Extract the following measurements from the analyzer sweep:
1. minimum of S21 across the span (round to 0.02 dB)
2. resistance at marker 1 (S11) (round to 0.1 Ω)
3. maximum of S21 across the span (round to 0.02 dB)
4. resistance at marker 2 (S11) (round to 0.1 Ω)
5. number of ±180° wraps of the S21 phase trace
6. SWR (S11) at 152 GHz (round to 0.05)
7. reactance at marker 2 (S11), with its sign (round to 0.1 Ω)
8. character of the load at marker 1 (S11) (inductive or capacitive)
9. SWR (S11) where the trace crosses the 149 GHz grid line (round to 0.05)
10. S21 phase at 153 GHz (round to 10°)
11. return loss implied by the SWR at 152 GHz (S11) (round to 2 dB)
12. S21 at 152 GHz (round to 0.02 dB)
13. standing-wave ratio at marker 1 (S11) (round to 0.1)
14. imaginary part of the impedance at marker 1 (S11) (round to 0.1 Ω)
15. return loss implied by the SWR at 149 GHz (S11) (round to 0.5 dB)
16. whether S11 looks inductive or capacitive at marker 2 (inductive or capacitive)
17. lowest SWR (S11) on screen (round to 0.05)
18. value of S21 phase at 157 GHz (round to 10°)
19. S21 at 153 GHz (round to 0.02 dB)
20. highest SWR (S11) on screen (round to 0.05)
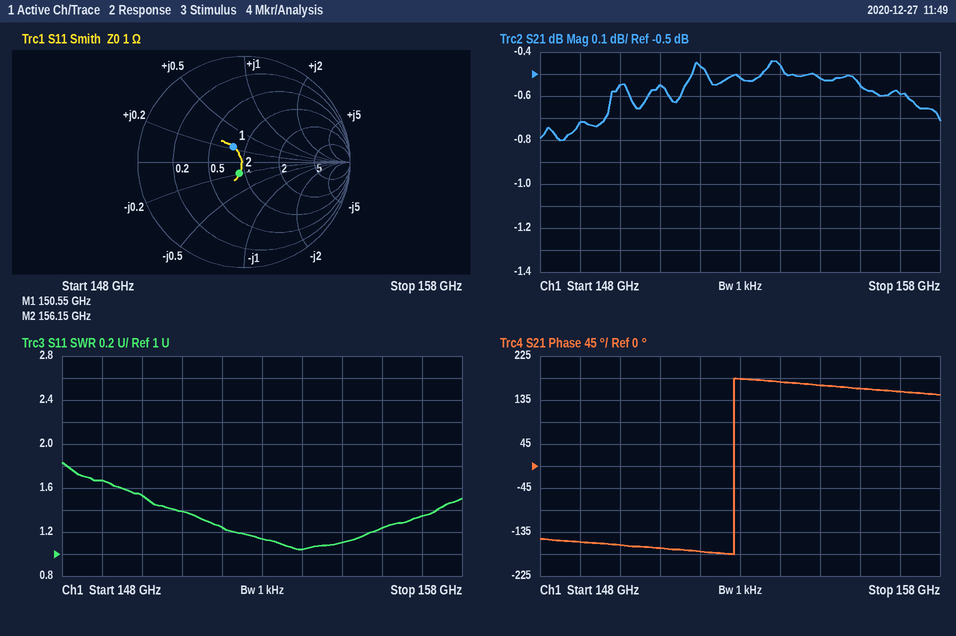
-0.80 dB
0.8 Ω
-0.44 dB
0.9 Ω
1
1.25
-0.2 Ω
inductive
1.65
180°
20 dB
-0.46 dB
1.4
+0.2 Ω
12.0 dB
capacitive
1.05
150°
-0.52 dB
1.85
